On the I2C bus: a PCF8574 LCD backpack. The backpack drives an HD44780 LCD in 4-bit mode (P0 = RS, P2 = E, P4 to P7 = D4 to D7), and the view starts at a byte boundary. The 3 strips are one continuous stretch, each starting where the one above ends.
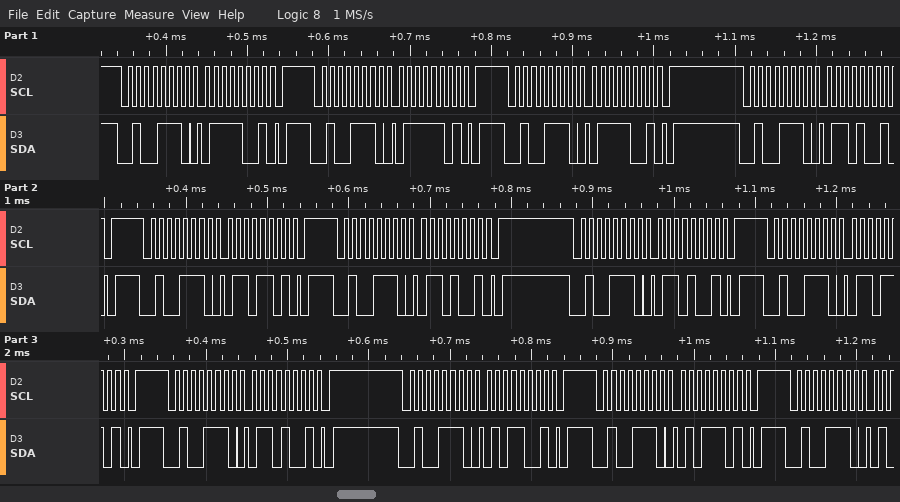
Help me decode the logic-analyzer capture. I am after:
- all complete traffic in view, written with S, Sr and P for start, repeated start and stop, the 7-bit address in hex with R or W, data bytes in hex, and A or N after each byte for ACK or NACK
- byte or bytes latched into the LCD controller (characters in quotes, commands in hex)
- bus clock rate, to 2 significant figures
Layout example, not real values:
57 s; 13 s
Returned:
S 27W A 79 A P S 27W A 7D A P S 27W A 79 A P S 27W A 69 A P S 27W A 6D A P S 27W A 69 A P S 27W A 69 A P S 27W A 6D A P S 27W A 69 A P S 27W A 59 A P S 27W A 5D A P S 27W A; 'v'; 100 kHz
